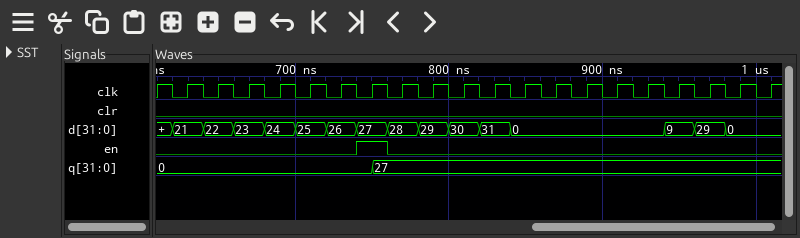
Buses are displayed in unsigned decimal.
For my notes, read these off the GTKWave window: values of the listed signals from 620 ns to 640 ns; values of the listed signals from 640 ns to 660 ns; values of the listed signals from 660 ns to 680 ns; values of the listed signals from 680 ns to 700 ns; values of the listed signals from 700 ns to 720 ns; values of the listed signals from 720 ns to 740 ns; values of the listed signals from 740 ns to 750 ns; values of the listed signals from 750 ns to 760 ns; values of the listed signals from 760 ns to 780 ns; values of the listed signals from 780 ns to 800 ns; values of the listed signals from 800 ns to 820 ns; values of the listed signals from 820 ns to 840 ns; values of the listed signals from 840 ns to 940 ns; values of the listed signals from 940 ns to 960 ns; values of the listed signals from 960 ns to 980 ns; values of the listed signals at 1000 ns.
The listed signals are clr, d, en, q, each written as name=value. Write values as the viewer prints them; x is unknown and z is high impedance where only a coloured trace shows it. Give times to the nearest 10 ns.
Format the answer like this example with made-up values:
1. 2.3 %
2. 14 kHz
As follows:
1. clr=0, d=21, en=0, q=0
2. clr=0, d=22, en=0, q=0
3. clr=0, d=23, en=0, q=0
4. clr=0, d=24, en=0, q=0
5. clr=0, d=25, en=0, q=0
6. clr=0, d=26, en=0, q=0
7. clr=0, d=27, en=1, q=0
8. clr=0, d=27, en=1, q=27
9. clr=0, d=28, en=0, q=27
10. clr=0, d=29, en=0, q=27
11. clr=0, d=30, en=0, q=27
12. clr=0, d=31, en=0, q=27
13. clr=0, d=0, en=0, q=27
14. clr=0, d=9, en=0, q=27
15. clr=0, d=29, en=0, q=27
16. clr=0, d=0, en=0, q=27
